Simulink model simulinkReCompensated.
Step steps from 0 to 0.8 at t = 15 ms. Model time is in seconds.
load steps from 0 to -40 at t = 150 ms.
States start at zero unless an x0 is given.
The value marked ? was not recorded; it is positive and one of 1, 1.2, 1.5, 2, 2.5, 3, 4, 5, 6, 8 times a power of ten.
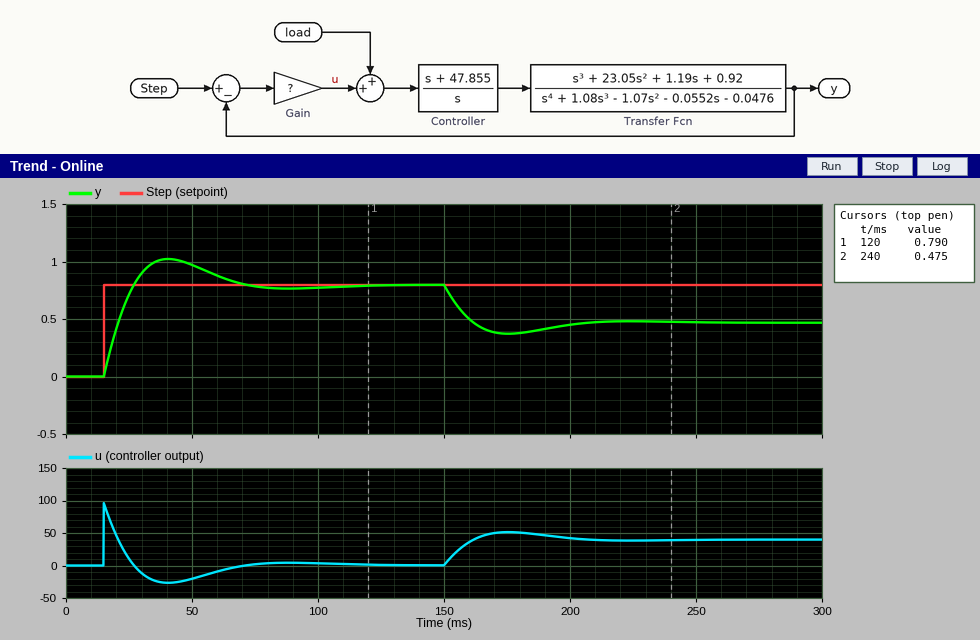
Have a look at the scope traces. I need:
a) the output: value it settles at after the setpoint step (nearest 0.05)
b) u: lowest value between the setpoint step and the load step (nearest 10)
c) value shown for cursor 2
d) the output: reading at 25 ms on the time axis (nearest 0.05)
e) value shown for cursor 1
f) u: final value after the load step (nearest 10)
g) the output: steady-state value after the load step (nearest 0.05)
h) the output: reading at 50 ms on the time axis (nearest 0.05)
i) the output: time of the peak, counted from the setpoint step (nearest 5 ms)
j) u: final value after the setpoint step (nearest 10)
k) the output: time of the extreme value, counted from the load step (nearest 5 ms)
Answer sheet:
0.80
-30
0.475
0.70
0.790
40
0.45
0.95
25 ms
0
25 ms
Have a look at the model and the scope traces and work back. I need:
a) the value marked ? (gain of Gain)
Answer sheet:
120
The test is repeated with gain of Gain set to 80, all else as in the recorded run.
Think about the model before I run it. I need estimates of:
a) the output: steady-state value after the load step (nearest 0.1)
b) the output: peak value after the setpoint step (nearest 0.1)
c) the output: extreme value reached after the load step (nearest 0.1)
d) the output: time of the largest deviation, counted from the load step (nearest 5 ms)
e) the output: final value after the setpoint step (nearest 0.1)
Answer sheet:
0.3
1.1
0.1
35 ms
0.8
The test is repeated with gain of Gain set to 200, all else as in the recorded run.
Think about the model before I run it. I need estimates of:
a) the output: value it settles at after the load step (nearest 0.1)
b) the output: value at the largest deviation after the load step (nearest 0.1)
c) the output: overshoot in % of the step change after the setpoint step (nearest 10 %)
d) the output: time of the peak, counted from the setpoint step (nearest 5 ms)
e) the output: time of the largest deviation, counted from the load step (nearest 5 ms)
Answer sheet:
0.6
0.6
20 %
20 ms
20 ms
